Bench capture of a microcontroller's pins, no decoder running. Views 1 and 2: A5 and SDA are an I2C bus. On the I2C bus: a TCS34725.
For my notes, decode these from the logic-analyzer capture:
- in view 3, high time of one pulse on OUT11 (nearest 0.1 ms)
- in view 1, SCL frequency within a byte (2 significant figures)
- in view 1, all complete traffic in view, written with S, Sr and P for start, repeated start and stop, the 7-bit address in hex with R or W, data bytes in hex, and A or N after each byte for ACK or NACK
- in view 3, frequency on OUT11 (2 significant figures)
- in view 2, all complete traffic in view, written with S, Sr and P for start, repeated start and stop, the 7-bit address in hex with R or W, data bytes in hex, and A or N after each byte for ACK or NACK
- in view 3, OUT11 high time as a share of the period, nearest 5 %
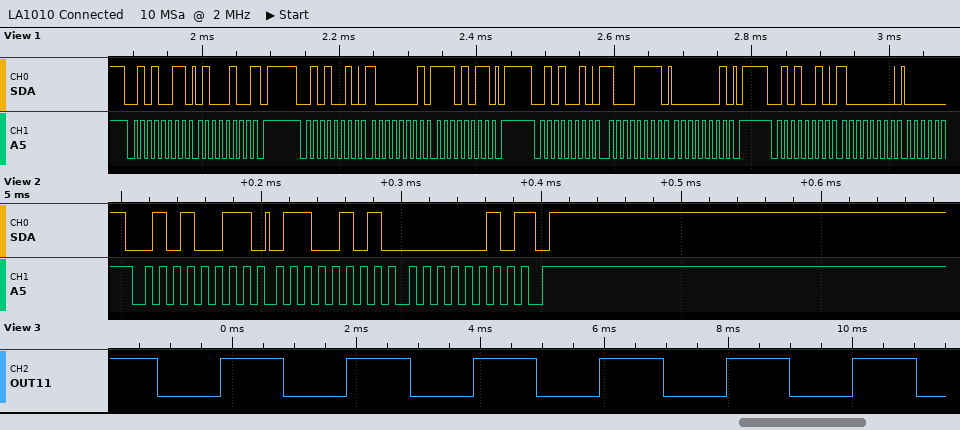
1.0 ms
100 kHz
S 29R A 44 N P S 29W A 81 A EB A P S 29W A 8F A 01 A P S 29W A 80 A
490 Hz
S 29R A 65 A 02 N P
50 %
